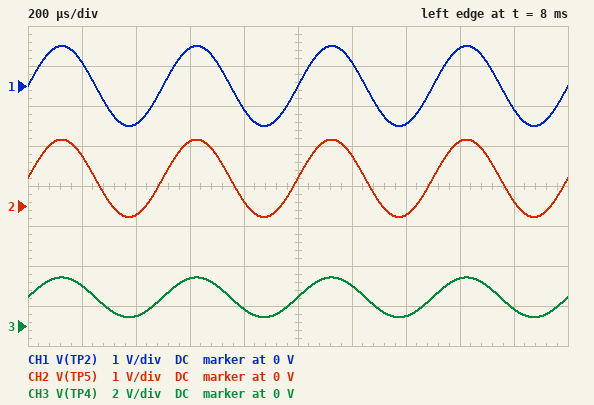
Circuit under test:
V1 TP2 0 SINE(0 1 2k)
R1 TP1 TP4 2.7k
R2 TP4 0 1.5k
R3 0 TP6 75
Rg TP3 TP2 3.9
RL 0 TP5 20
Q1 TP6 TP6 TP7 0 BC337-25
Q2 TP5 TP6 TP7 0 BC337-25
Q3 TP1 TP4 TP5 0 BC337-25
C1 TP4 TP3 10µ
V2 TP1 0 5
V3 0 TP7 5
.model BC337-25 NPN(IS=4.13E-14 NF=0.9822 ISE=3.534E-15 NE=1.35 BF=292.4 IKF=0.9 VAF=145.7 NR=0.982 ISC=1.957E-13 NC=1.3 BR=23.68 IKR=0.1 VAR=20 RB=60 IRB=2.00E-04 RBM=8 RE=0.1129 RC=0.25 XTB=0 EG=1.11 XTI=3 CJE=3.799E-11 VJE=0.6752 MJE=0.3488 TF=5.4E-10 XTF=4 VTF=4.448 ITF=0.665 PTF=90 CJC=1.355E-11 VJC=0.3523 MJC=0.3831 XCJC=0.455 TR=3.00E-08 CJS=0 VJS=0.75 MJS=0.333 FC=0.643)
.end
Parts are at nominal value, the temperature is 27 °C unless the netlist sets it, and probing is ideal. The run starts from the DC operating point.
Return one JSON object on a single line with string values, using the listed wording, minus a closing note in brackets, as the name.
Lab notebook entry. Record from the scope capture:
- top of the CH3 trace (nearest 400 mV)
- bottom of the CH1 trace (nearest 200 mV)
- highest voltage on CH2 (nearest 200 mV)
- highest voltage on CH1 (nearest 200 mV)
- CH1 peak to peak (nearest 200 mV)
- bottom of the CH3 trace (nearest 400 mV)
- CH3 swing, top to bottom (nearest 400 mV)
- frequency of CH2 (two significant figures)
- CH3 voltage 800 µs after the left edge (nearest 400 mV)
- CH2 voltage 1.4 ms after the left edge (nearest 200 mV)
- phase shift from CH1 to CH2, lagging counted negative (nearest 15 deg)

{"top of the CH3 trace": "2.4 V", "bottom of the CH1 trace": "-1.0 V", "highest voltage on CH2": "1.6 V", "highest voltage on CH1": "1.0 V", "CH1 peak to peak": "2.0 V", "bottom of the CH3 trace": "400 mV", "CH3 swing, top to bottom": "2.0 V", "frequency of CH2": "2.0 kHz", "CH3 voltage 800 µs after the left edge": "800 mV", "CH2 voltage 1.4 ms after the left edge": "-200 mV", "phase shift from CH1 to CH2, lagging counted negative": "0 deg"}
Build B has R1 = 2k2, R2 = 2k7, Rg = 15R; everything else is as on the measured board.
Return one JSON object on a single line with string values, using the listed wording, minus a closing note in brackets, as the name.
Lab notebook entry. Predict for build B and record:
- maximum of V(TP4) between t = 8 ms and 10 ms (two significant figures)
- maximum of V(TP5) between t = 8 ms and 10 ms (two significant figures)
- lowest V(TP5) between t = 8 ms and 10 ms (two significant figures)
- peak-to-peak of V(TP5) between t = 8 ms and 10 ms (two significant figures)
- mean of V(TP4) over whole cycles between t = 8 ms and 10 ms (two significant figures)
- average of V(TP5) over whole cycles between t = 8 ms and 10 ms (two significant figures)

{"maximum of V(TP4) between t = 8 ms and 10 ms": "3.1 V", "maximum of V(TP5) between t = 8 ms and 10 ms": "2.3 V", "lowest V(TP5) between t = 8 ms and 10 ms": "410 mV", "peak-to-peak of V(TP5) between t = 8 ms and 10 ms": "1.9 V", "mean of V(TP4) over whole cycles between t = 8 ms and 10 ms": "2.1 V", "average of V(TP5) over whole cycles between t = 8 ms and 10 ms": "1.4 V"}
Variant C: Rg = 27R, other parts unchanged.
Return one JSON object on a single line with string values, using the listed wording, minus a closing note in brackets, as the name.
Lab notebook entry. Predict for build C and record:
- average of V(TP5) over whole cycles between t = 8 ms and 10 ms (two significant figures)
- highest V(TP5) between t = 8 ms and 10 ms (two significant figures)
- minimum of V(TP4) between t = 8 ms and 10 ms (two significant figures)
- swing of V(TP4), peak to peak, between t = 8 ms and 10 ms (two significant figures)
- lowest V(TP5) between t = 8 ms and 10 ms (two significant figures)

{"average of V(TP5) over whole cycles between t = 8 ms and 10 ms": "690 mV", "highest V(TP5) between t = 8 ms and 10 ms": "1.6 V", "minimum of V(TP4) between t = 8 ms and 10 ms": "470 mV", "swing of V(TP4), peak to peak, between t = 8 ms and 10 ms": "1.9 V", "lowest V(TP5) between t = 8 ms and 10 ms": "-250 mV"}
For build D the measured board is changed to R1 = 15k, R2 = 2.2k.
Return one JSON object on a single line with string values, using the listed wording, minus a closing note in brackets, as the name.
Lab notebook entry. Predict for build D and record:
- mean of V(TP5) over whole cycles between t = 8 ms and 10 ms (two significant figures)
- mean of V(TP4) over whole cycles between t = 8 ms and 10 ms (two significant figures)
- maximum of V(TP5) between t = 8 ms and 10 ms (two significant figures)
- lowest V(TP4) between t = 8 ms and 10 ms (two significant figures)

{"mean of V(TP5) over whole cycles between t = 8 ms and 10 ms": "-330 mV", "mean of V(TP4) over whole cycles between t = 8 ms and 10 ms": "350 mV", "maximum of V(TP5) between t = 8 ms and 10 ms": "600 mV", "lowest V(TP4) between t = 8 ms and 10 ms": "-650 mV"}
